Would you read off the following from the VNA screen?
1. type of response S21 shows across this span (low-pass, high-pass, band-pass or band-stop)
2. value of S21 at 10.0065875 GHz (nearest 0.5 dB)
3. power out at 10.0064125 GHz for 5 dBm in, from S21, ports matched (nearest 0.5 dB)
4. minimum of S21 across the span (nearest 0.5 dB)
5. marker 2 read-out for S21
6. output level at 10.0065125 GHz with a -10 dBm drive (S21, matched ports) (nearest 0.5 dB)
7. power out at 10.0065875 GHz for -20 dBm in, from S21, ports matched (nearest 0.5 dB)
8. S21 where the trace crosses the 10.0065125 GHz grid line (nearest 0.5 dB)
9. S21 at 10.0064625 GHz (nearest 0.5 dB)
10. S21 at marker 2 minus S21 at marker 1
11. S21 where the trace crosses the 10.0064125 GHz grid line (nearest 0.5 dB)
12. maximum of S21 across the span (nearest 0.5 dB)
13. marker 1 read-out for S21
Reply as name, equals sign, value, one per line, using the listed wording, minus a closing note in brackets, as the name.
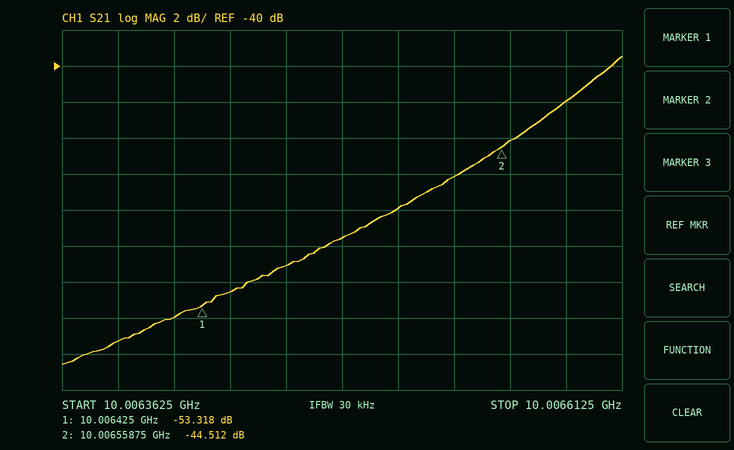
type of response S21 shows across this span = high-pass
value of S21 at 10.0065875 GHz = -42.0 dB
power out at 10.0064125 GHz for 5 dBm in, from S21, ports matched = -49.0 dBm
minimum of S21 across the span = -56.5 dB
marker 2 read-out for S21 = -44.512 dB
output level at 10.0065125 GHz with a -10 dBm drive (S21, matched ports) = -58.0 dBm
power out at 10.0065875 GHz for -20 dBm in, from S21, ports matched = -62.0 dBm
S21 where the trace crosses the 10.0065125 GHz grid line = -48.0 dB
S21 at 10.0064625 GHz = -51.0 dB
S21 at marker 2 minus S21 at marker 1 = 8.806 dB
S21 where the trace crosses the 10.0064125 GHz grid line = -54.0 dB
maximum of S21 across the span = -39.5 dB
marker 1 read-out for S21 = -53.318 dB
